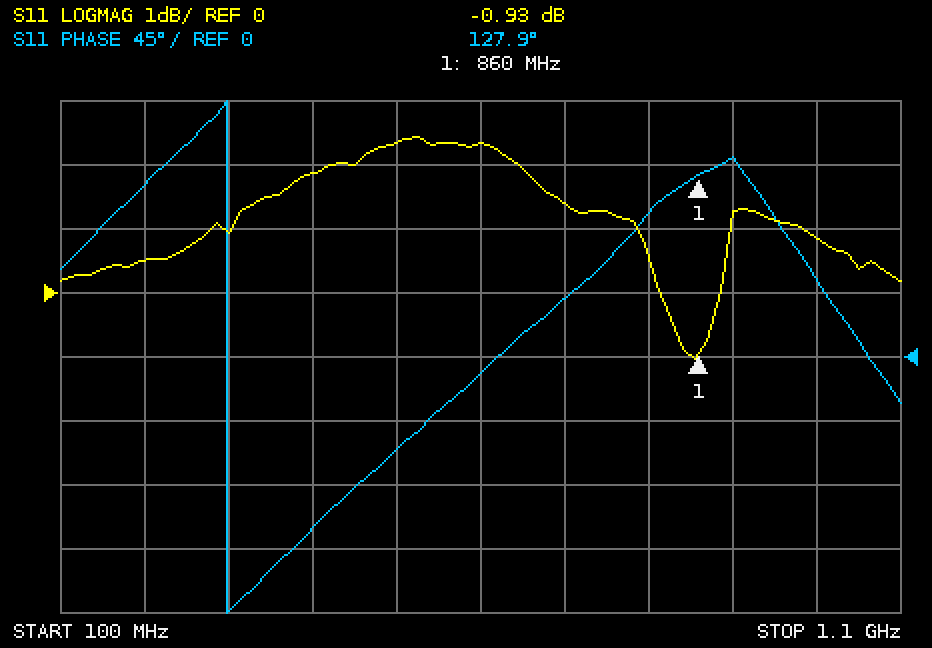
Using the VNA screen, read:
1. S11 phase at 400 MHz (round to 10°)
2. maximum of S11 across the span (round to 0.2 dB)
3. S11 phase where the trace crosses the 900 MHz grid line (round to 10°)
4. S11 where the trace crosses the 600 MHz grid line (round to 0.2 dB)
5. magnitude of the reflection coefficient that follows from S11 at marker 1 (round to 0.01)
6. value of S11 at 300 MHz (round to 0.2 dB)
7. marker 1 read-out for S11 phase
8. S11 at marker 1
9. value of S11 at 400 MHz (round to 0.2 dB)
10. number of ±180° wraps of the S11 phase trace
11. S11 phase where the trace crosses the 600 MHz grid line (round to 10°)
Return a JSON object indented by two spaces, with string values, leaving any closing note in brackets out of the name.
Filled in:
{
  "S11 phase at 400 MHz": "-120°",
  "maximum of S11 across the span": "2.4 dB",
  "S11 phase where the trace crosses the 900 MHz grid line": "140°",
  "S11 where the trace crosses the 600 MHz grid line": "2.4 dB",
  "magnitude of the reflection coefficient that follows from S11 at marker 1": "0.90",
  "value of S11 at 300 MHz": "1.0 dB",
  "marker 1 read-out for S11 phase": "127.9°",
  "S11 at marker 1": "-0.93 dB",
  "value of S11 at 400 MHz": "1.8 dB",
  "number of ±180° wraps of the S11 phase trace": "1",
  "S11 phase where the trace crosses the 600 MHz grid line": "-10°"
}
